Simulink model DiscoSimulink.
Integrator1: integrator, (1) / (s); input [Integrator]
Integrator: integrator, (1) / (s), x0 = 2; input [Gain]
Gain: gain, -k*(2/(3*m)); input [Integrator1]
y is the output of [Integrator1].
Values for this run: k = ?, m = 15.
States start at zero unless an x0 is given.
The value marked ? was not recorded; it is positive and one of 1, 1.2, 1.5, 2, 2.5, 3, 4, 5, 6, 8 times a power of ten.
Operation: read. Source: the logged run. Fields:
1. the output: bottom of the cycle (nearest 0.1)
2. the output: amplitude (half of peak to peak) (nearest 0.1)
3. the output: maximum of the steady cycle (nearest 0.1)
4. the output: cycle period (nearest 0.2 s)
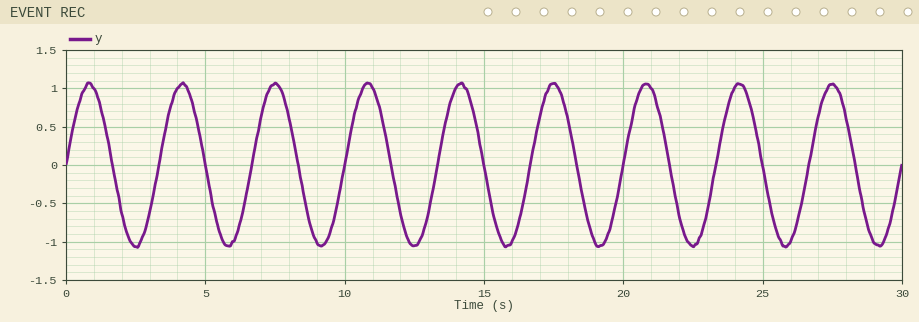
-1.1
1.1
1.1
3.4 s
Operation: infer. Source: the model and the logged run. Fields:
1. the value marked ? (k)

80
